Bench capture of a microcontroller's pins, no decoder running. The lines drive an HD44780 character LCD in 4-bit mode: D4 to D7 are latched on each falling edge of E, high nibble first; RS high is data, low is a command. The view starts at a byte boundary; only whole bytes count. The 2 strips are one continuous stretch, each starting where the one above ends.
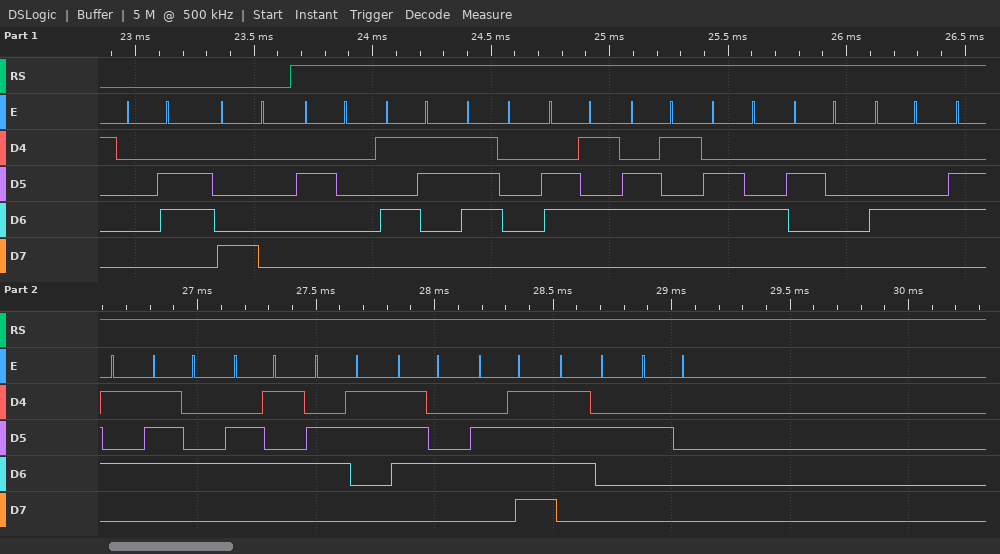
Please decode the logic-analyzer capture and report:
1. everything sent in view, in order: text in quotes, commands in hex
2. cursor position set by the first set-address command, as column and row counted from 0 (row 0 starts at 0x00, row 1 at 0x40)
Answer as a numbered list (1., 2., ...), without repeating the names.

1. 0x06 0x80 " Speed Detector "
2. column 0, row 0
